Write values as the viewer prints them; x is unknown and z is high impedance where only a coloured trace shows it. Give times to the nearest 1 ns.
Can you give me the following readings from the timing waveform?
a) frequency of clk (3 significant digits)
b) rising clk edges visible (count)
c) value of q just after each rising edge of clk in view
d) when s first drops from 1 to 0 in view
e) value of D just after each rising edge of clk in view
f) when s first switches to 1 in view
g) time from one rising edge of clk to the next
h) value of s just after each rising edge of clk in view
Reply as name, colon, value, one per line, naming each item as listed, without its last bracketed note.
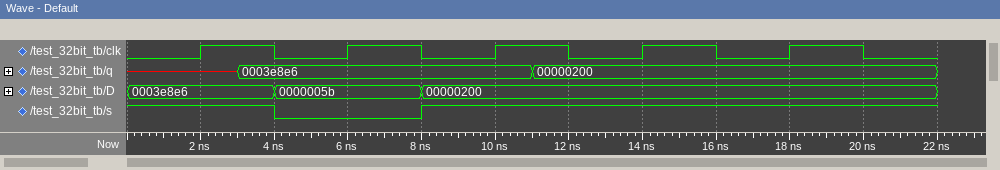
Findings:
frequency of clk: 250 MHz
rising clk edges visible: 5
value of q just after each rising edge of clk in view: x, 0003e8e6, 0003e8e6, 00000200, 00000200
when s first drops from 1 to 0 in view: 4 ns
value of D just after each rising edge of clk in view: 0003e8e6, 0000005b, 00000200, 00000200, 00000200
when s first switches to 1 in view: 8 ns
time from one rising edge of clk to the next: 4 ns
value of s just after each rising edge of clk in view: 1 0 1 1 1
